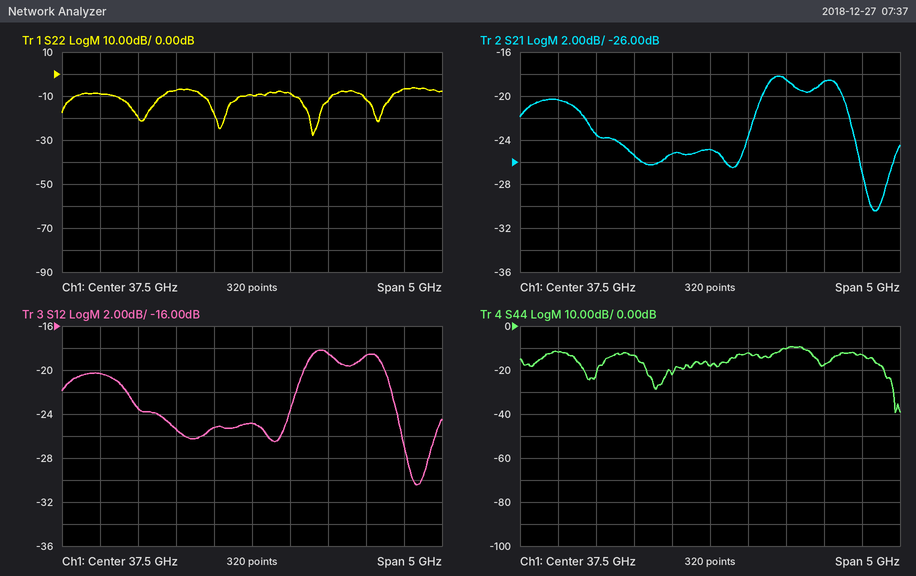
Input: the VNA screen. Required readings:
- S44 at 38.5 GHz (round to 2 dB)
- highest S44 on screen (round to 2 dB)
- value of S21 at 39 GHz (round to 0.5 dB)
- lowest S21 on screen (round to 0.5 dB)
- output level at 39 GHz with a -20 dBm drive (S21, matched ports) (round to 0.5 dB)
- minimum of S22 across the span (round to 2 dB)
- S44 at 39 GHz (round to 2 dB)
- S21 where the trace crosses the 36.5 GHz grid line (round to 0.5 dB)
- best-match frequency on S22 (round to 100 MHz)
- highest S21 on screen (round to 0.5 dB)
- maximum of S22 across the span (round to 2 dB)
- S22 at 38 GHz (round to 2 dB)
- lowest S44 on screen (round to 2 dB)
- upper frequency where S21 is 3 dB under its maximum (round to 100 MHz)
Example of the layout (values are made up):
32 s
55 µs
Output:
-10 dB
-10 dB
-18.5 dB
-30.5 dB
-38.5 dBm
-28 dB
-18 dB
-25.5 dB
38.3 GHz
-18.0 dB
-6 dB
-8 dB
-40 dB
39.3 GHz
